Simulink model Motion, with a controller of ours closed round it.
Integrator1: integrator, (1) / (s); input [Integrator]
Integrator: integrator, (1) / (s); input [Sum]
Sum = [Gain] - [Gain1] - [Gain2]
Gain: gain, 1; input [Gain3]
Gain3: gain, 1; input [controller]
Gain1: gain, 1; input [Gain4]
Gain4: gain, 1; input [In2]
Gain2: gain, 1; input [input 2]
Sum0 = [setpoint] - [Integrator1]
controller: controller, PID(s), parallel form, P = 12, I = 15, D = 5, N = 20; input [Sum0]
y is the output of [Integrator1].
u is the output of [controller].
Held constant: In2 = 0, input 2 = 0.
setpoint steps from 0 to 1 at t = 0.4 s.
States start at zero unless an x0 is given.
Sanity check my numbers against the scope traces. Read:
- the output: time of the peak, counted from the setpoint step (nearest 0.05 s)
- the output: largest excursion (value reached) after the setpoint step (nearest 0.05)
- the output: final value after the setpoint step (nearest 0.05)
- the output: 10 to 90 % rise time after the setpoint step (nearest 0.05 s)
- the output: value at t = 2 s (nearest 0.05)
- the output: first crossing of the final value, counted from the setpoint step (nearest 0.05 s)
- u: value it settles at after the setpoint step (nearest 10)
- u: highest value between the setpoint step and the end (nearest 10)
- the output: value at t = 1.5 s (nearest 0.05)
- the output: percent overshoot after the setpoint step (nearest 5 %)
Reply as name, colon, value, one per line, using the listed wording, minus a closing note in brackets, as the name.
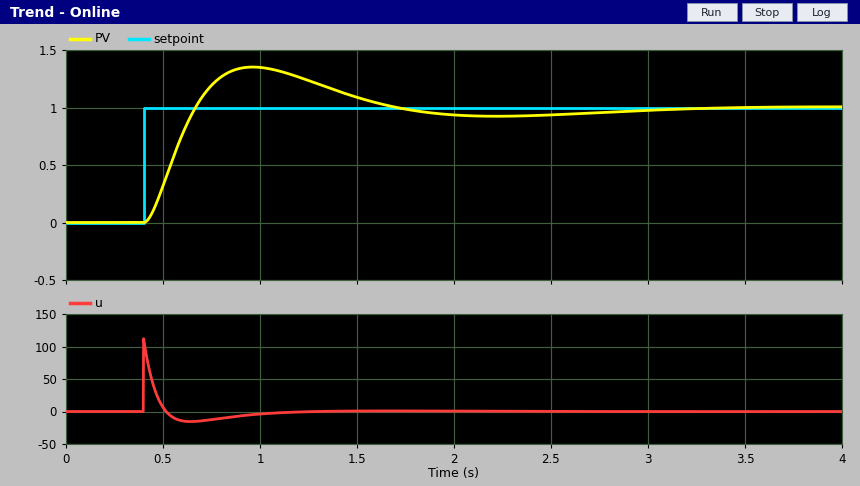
the output: time of the peak, counted from the setpoint step: 0.55 s
the output: largest excursion (value reached) after the setpoint step: 1.35
the output: final value after the setpoint step: 1.00
the output: 10 to 90 % rise time after the setpoint step: 0.20 s
the output: value at t = 2 s: 0.95
the output: first crossing of the final value, counted from the setpoint step: 0.25 s
u: value it settles at after the setpoint step: 0
u: highest value between the setpoint step and the end: 110
the output: value at t = 1.5 s: 1.10
the output: percent overshoot after the setpoint step: 35 %
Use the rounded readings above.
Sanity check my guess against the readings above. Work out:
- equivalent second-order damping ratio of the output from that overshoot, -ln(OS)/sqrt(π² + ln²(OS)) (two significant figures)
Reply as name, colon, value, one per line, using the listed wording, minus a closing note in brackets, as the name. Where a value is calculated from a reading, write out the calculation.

equivalent second-order damping ratio of the output from that overshoot, -ln(OS)/sqrt(π² + ln²(OS)): ln(0.35) = -1.050; 1.050 / sqrt(9.870 + 1.102) = 0.32
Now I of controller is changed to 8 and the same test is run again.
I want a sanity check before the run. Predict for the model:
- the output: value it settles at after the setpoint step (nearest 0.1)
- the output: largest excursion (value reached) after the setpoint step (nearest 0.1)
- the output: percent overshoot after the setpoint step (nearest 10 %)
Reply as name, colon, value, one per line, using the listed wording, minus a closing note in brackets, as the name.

the output: value it settles at after the setpoint step: 1.0
the output: largest excursion (value reached) after the setpoint step: 1.3
the output: percent overshoot after the setpoint step: 30 %
